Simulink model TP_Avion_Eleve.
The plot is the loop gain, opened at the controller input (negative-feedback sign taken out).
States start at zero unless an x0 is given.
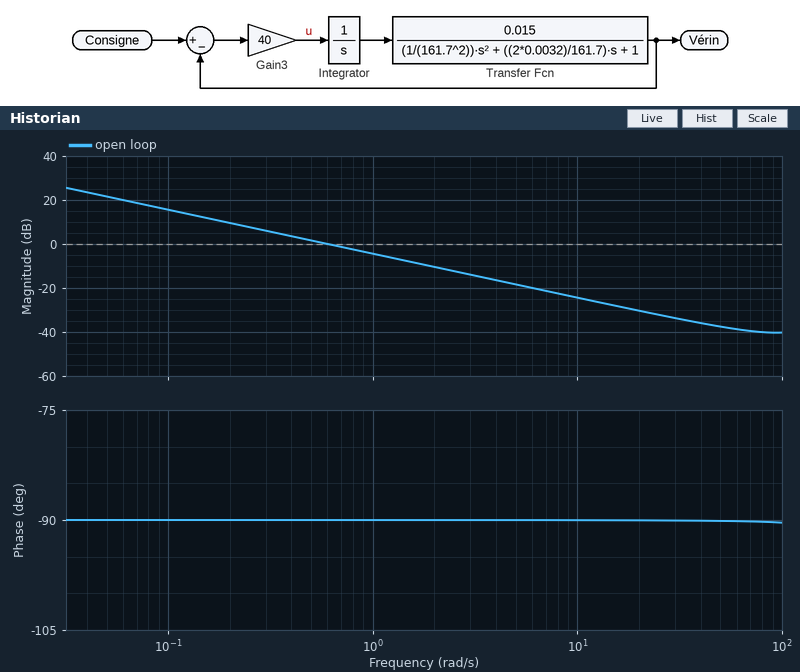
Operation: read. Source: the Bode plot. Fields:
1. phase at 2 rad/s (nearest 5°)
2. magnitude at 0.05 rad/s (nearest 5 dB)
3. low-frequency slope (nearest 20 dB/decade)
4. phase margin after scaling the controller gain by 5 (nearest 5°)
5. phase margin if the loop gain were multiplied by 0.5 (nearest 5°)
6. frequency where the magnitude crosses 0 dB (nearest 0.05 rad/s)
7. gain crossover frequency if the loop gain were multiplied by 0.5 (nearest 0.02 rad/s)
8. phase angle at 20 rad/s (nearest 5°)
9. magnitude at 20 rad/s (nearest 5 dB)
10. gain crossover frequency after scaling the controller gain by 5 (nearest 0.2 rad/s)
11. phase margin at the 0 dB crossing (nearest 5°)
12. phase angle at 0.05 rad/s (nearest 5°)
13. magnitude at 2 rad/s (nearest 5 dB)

-90°
20 dB
-20 dB/decade
90°
90°
0.60 rad/s
0.30 rad/s
-90°
-30 dB
3.0 rad/s
90°
-90°
-10 dB
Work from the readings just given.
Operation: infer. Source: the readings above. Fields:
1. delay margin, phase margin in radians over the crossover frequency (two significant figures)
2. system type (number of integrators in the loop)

2.6 s
1
